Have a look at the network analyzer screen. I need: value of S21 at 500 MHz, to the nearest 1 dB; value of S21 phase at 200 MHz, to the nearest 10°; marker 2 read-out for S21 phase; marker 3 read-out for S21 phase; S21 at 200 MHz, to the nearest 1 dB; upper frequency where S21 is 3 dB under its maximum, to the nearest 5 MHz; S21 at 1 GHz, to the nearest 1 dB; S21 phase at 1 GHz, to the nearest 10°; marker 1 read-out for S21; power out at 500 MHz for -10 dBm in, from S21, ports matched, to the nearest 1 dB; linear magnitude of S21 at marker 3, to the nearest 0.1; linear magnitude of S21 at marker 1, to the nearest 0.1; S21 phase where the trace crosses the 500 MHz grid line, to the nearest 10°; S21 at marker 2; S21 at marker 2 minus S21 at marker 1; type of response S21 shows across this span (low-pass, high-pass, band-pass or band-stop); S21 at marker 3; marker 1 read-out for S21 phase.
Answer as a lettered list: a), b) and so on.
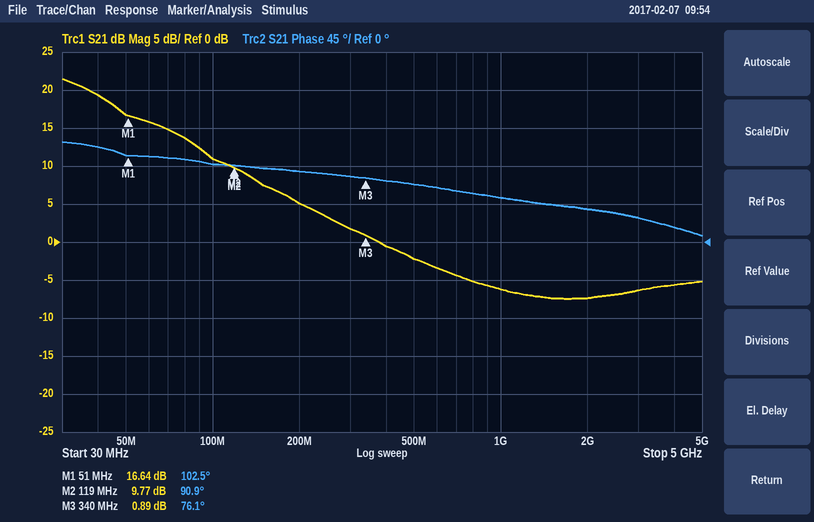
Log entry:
a) -2 dB
b) 80°
c) 90.9°
d) 76.1°
e) 5 dB
f) 45 MHz
g) -6 dB
h) 50°
i) 16.64 dB
j) -12 dBm
k) 1.1
l) 6.8
m) 70°
n) 9.77 dB
o) -6.87 dB
p) low-pass
q) 0.89 dB
r) 102.5°
